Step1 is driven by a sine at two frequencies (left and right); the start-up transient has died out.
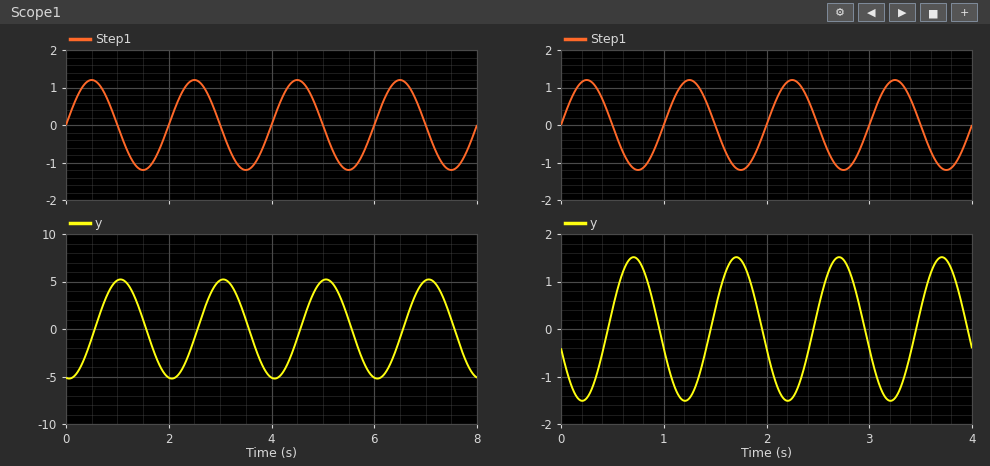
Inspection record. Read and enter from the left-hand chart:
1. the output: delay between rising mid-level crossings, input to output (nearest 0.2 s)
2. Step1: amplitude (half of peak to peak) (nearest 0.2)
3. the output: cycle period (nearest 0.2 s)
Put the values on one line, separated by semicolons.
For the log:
0.6 s; 1.2; 2.0 s
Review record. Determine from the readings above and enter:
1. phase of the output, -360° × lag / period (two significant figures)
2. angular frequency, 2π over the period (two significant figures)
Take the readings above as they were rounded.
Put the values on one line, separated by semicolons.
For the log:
-110°; 3.1 rad/s
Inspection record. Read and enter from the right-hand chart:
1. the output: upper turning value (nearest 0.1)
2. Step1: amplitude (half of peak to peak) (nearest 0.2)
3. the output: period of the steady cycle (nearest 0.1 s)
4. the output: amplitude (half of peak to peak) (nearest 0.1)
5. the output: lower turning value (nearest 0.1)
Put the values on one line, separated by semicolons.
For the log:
1.5; 1.2; 1.0 s; 1.5; -1.5
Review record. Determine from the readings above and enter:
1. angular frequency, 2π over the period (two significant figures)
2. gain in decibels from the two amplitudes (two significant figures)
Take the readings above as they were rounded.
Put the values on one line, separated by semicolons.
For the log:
6.3 rad/s; 1.9 dB
